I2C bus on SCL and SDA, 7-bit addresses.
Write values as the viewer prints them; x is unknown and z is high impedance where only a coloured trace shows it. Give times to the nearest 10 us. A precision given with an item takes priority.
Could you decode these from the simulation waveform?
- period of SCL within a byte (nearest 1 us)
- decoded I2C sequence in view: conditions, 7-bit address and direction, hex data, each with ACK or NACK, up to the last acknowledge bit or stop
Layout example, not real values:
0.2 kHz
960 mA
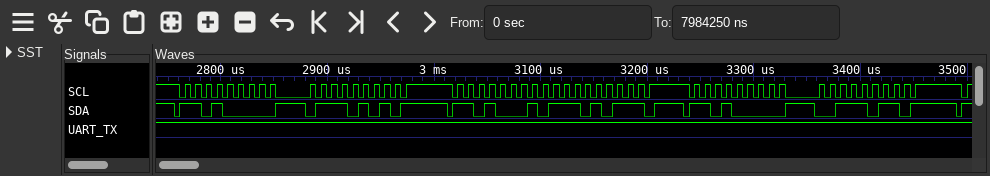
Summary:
10 us
start, address 68 write ACK, 75 ACK, repeated start, address 68 read ACK, EB NACK, stop, start, address 68 write ACK, 3B ACK
